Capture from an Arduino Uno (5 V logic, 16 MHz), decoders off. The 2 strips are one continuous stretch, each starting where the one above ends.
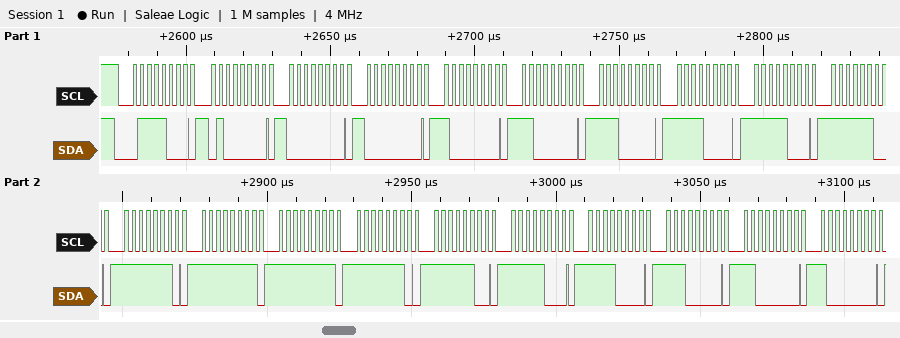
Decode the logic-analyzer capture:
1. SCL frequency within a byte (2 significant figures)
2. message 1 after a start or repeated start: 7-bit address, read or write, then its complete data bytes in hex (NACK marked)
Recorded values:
400 kHz
0x3C write: 40 00 00 80 C0 E0 F0 F8 FC FE FF FF FE FC F8 F0 E0 C0 80
